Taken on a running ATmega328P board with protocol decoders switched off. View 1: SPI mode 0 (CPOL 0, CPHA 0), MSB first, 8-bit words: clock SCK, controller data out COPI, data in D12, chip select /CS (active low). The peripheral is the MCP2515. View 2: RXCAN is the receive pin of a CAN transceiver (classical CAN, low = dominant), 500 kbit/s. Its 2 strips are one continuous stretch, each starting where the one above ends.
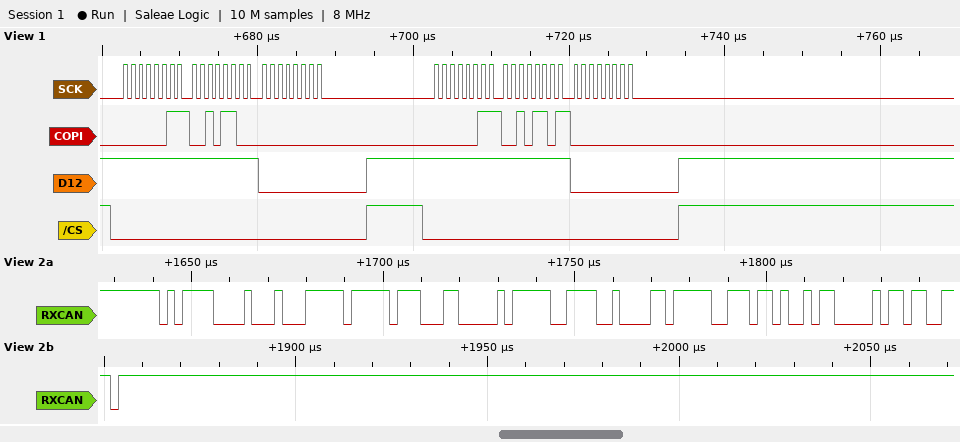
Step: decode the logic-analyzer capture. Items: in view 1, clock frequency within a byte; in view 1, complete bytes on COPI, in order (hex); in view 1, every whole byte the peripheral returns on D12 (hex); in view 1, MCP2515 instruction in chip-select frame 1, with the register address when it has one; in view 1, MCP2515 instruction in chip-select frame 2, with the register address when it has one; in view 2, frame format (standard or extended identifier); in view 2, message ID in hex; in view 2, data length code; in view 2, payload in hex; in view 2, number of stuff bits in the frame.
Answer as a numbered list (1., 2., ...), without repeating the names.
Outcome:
1. 1 MHz
2. 0x03 0x2C 0x00 0x03 0x2D 0x00
3. 0xFF 0xFF 0x00 0xFF 0xFF 0x00
4. READ 0x2C
5. READ 0x2D
6. standard
7. 0x5E1
8. 8
9. FF F8 C0 FB C8 6F BB 4B
10. 6
